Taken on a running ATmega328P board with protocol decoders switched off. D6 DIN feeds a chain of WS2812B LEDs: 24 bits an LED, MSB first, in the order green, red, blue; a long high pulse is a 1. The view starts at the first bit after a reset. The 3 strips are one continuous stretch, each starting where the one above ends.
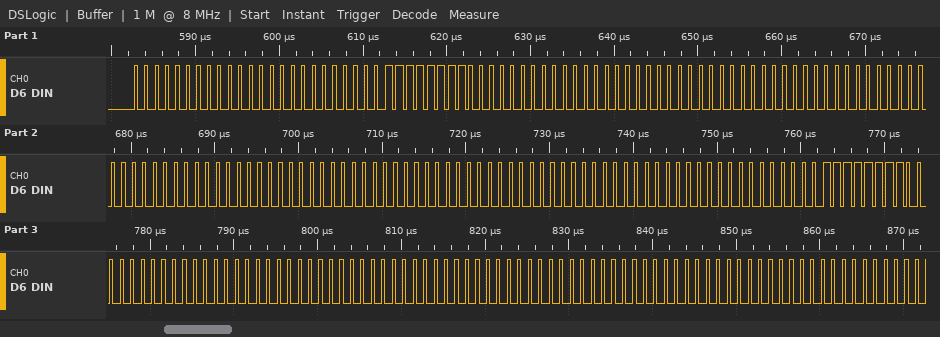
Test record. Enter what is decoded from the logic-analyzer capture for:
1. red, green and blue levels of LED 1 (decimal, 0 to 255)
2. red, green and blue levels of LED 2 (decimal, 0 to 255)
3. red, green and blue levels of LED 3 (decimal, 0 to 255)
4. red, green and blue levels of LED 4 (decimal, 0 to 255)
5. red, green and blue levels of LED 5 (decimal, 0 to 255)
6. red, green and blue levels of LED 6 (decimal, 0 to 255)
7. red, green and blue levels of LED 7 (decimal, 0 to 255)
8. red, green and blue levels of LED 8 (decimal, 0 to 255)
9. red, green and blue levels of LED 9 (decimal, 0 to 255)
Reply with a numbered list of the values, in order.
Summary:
1. 0, 0, 0
2. 0, 255, 0
3. 0, 0, 0
4. 0, 0, 0
5. 0, 0, 0
6. 0, 0, 0
7. 0, 255, 0
8. 0, 0, 0
9. 0, 0, 0
